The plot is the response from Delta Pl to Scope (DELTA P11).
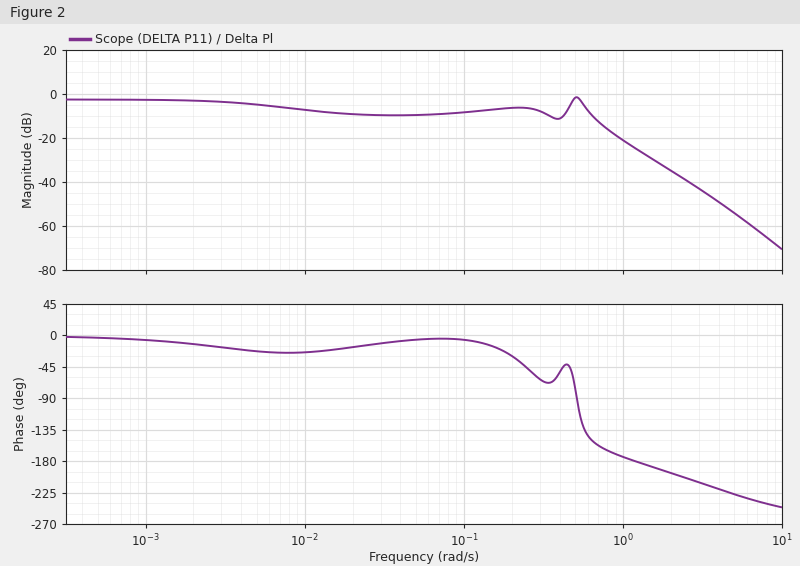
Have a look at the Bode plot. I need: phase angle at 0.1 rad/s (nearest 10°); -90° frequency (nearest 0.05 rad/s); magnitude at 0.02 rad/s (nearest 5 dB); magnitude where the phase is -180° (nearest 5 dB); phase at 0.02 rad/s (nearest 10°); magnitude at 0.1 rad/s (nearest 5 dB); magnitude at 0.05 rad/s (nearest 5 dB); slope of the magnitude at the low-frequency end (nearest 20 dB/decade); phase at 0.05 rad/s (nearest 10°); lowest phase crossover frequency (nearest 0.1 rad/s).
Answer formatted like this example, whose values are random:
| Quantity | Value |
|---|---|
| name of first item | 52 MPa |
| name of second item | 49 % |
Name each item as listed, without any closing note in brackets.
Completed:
| Quantity | Value |
|---|---|
| phase angle at 0.1 rad/s | -10° |
| -90° frequency | 0.50 rad/s |
| magnitude at 0.02 rad/s | -10 dB |
| magnitude where the phase is -180° | -25 dB |
| phase at 0.02 rad/s | -20° |
| magnitude at 0.1 rad/s | -10 dB |
| magnitude at 0.05 rad/s | -10 dB |
| slope of the magnitude at the low-frequency end | 0 dB/decade |
| phase at 0.05 rad/s | -10° |
| lowest phase crossover frequency | 1.2 rad/s |
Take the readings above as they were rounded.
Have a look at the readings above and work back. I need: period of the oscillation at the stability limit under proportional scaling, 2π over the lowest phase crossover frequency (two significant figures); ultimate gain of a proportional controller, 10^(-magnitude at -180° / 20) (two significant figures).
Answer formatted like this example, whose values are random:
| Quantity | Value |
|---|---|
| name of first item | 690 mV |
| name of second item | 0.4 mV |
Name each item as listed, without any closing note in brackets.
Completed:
| Quantity | Value |
|---|---|
| period of the oscillation at the stability limit under proportional scaling, 2π over the lowest phase crossover frequency | 5.2 s |
| ultimate gain of a proportional controller, 10^(-magnitude at -180° / 20) | 18 |
